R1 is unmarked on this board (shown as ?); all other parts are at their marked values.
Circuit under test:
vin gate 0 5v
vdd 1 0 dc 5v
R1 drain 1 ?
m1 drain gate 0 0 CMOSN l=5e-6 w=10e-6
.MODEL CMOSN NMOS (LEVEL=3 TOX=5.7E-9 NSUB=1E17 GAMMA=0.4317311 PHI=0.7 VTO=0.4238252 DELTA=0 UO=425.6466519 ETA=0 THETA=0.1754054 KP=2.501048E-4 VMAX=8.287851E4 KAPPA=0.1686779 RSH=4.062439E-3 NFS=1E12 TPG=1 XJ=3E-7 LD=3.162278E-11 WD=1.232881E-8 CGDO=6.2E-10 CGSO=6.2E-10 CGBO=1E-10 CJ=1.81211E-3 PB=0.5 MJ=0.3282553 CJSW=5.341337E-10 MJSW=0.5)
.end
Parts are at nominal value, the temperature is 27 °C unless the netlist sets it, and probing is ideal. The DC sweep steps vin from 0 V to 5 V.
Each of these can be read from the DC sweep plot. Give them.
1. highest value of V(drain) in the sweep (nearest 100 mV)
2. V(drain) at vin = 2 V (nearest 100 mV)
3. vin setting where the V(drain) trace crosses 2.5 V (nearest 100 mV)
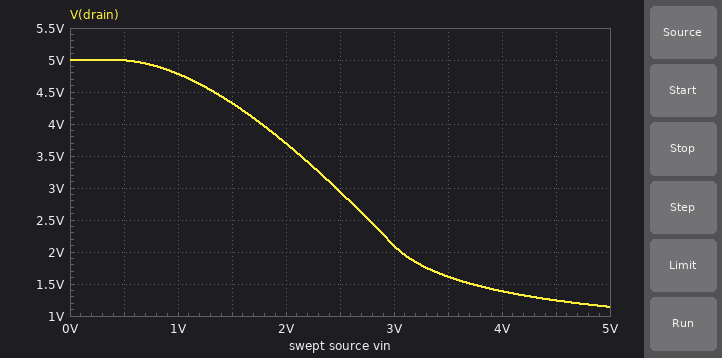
5.0 V
3.7 V
2.8 V
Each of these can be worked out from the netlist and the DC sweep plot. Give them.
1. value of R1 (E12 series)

3.3 kΩ
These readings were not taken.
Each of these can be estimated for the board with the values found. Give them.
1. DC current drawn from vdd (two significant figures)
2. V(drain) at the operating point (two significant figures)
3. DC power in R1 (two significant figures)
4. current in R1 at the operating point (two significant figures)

1.2 mA
1.1 V
4.5 mW
1.2 mA
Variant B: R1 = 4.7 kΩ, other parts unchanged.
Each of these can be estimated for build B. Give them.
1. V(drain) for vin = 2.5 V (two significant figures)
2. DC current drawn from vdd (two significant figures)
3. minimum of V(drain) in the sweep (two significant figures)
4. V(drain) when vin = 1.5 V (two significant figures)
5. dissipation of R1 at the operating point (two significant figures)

2.1 V
890 µA
820 mV
4.0 V
3.7 mW
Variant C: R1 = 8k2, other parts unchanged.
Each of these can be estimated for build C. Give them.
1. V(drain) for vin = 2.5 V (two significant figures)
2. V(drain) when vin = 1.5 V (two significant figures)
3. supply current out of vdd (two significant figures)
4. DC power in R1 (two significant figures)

930 mV
3.3 V
550 µA
2.5 mW
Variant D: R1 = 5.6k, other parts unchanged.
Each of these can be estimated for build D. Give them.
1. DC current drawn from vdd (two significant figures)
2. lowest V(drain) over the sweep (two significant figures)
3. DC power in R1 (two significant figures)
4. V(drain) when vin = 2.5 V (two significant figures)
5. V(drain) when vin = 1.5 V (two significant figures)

770 µA
690 mV
3.3 mW
1.6 V
3.9 V
